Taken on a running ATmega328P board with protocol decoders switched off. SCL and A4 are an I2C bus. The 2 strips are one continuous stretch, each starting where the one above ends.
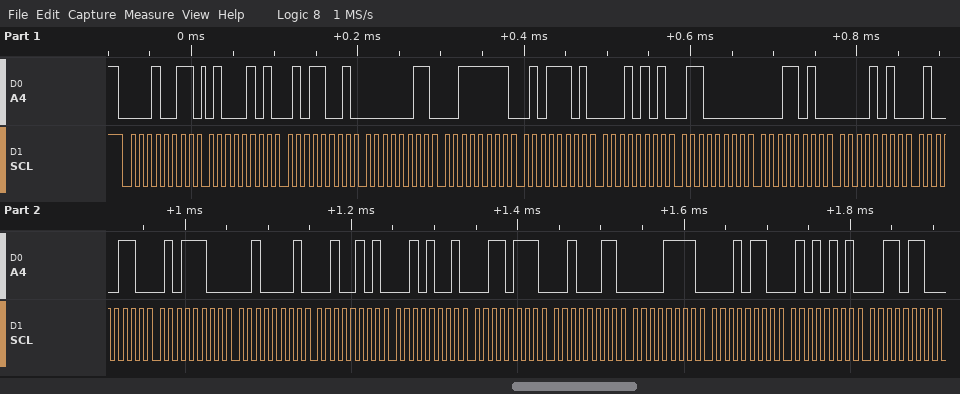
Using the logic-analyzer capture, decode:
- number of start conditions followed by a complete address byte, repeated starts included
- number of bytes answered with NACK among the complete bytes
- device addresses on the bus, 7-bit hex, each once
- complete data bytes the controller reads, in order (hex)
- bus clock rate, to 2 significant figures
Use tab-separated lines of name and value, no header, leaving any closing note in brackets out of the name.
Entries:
number of start conditions followed by a complete address byte, repeated starts included	1
number of bytes answered with NACK among the complete bytes	0
device addresses on the bus, 7-bit hex, each once	0x09
complete data bytes the controller reads, in order	45 59 03 3F 5D 15 60 1A 0A 46 5C 21 25 29 37 23 0F 16 55 36
bus clock rate, to 2 significant figures	100 kHz
